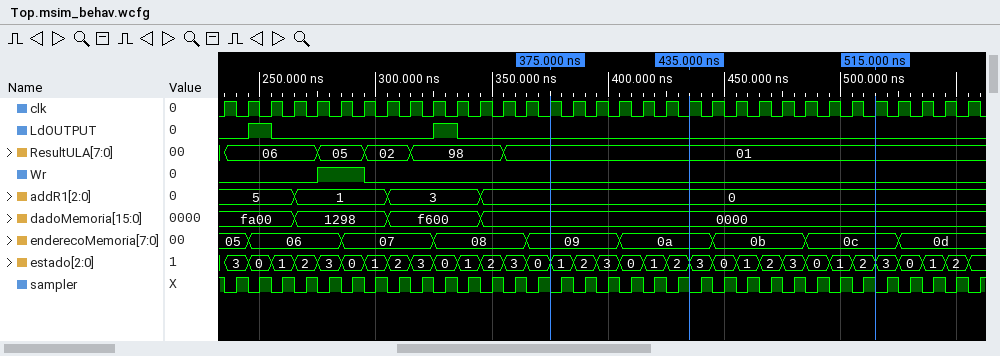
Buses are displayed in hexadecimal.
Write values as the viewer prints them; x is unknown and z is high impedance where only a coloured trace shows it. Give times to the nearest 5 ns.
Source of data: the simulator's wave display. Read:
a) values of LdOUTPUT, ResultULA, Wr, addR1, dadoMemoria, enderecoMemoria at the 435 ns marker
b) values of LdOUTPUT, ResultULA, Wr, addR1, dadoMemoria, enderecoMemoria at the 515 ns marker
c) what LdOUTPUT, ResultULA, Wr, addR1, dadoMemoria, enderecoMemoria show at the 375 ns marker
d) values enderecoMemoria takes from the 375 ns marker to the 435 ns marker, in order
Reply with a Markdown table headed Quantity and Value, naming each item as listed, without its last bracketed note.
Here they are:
| Quantity | Value |
|---|---|
| values of LdOUTPUT, ResultULA, Wr, addR1, dadoMemoria, enderecoMemoria at the 435 ns marker | LdOUTPUT=0, ResultULA=01, Wr=0, addR1=0, dadoMemoria=0000, enderecoMemoria=0a |
| values of LdOUTPUT, ResultULA, Wr, addR1, dadoMemoria, enderecoMemoria at the 515 ns marker | LdOUTPUT=0, ResultULA=01, Wr=0, addR1=0, dadoMemoria=0000, enderecoMemoria=0c |
| what LdOUTPUT, ResultULA, Wr, addR1, dadoMemoria, enderecoMemoria show at the 375 ns marker | LdOUTPUT=0, ResultULA=01, Wr=0, addR1=0, dadoMemoria=0000, enderecoMemoria=09 |
| values enderecoMemoria takes from the 375 ns marker to the 435 ns marker, in order | 09, 0a |
